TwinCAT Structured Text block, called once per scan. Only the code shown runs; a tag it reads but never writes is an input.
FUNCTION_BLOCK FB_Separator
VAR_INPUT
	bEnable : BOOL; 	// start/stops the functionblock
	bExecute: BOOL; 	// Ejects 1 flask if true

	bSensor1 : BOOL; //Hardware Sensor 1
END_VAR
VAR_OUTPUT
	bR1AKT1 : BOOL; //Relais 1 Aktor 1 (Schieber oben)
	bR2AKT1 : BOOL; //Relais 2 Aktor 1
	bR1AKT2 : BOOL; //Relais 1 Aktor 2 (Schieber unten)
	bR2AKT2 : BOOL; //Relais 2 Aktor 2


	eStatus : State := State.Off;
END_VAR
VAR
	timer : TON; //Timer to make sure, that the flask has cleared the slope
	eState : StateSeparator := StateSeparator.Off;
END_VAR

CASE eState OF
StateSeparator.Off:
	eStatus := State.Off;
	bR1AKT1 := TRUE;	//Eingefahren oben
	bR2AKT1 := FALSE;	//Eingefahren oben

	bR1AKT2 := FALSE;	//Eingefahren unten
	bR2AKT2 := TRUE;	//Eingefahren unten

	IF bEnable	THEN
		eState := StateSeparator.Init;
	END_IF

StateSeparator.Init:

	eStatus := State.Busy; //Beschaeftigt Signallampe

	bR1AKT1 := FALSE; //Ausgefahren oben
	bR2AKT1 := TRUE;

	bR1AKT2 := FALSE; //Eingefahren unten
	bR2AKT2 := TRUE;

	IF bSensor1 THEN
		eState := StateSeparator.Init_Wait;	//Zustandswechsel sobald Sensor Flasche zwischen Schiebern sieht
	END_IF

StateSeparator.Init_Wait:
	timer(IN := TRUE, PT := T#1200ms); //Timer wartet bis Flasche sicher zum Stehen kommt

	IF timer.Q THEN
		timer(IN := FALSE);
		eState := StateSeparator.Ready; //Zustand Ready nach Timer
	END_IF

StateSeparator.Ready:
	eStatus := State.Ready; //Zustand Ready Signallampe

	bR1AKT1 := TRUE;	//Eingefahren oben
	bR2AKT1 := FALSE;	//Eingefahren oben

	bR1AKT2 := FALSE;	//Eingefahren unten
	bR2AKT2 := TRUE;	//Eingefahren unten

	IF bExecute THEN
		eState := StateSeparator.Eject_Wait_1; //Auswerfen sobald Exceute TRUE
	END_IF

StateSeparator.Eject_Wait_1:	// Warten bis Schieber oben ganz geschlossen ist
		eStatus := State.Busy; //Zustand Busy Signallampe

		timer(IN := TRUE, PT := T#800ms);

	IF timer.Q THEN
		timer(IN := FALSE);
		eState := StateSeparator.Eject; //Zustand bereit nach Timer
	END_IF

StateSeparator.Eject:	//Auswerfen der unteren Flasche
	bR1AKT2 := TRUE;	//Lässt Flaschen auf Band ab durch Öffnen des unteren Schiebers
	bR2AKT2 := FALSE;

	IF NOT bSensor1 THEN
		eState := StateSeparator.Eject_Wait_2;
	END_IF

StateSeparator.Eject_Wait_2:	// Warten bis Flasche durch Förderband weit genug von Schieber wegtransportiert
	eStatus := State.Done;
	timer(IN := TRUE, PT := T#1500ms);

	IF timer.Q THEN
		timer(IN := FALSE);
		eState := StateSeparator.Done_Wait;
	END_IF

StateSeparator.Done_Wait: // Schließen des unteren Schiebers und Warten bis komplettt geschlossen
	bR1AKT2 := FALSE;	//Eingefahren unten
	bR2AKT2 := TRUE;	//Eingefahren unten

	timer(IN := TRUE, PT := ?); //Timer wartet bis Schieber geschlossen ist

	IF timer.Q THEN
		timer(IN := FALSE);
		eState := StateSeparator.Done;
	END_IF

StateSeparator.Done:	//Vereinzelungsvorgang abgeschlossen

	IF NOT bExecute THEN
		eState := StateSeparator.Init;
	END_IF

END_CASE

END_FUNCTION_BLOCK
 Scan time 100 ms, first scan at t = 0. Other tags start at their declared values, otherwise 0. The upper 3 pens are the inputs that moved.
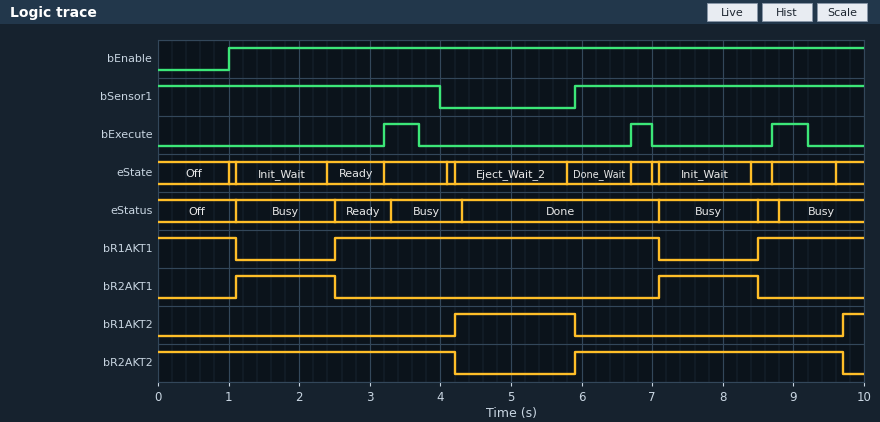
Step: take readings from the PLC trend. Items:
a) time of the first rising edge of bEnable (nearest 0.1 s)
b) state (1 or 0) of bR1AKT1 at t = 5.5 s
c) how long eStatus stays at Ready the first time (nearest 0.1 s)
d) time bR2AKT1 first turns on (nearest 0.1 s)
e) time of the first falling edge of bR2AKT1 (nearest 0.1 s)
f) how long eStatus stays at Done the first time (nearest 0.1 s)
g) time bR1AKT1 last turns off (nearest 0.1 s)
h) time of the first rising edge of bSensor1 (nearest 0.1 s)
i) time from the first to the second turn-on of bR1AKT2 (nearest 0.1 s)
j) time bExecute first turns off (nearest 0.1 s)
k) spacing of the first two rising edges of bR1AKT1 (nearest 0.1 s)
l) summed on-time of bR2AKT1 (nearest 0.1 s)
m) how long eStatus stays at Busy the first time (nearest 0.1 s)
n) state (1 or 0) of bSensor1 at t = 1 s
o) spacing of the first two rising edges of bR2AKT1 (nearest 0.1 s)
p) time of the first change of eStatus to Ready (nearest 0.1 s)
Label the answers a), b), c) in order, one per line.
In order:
a) 1.0 s
b) 1
c) 0.8 s
d) 1.1 s
e) 2.5 s
f) 2.8 s
g) 7.1 s
h) 5.9 s
i) 5.5 s
j) 3.7 s
k) 6.0 s
l) 2.8 s
m) 1.4 s
n) 1
o) 6.0 s
p) 2.5 s
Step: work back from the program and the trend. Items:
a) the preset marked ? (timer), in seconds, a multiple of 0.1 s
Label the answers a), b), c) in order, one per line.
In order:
a) 0.8 s
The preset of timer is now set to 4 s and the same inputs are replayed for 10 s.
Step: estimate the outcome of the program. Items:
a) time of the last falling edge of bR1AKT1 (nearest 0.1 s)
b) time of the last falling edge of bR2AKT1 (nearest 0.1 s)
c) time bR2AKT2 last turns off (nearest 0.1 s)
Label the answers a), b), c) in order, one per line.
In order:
a) 1.1 s
b) 2.5 s
c) 4.2 s
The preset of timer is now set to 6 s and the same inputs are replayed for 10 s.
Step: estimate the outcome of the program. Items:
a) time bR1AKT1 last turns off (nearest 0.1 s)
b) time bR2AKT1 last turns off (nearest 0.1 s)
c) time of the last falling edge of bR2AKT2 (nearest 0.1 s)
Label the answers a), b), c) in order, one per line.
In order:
a) 1.1 s
b) 2.5 s
c) 4.2 s
